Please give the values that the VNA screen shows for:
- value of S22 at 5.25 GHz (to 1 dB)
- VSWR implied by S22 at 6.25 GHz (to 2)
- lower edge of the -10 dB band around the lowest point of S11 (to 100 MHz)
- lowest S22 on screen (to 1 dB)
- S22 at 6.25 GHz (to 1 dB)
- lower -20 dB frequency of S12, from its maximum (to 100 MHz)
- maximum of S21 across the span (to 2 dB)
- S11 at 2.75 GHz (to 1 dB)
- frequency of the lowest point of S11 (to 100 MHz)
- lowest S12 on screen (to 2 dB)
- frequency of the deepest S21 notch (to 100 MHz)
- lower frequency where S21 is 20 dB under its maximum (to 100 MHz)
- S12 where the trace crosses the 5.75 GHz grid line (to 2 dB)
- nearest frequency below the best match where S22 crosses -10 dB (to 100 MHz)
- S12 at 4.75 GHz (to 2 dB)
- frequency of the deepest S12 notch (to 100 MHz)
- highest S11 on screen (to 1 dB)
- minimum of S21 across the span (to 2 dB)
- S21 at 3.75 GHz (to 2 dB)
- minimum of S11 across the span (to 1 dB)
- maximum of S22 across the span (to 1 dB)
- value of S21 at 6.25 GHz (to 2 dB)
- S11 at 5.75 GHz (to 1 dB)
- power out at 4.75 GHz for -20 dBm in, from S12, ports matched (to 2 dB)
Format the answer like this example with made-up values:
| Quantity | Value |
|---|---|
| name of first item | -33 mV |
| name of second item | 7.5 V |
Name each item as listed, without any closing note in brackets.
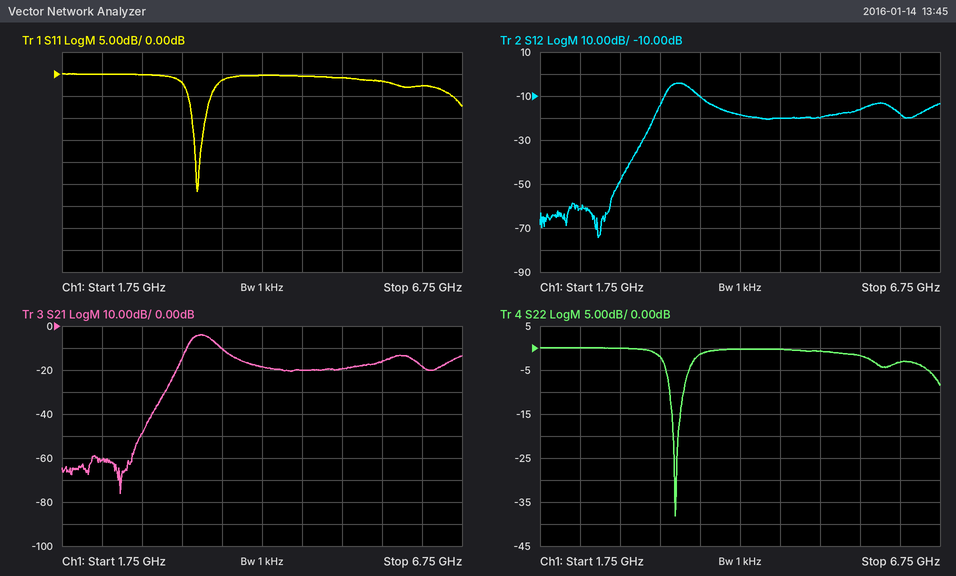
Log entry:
| Quantity | Value |
|---|---|
| value of S22 at 5.25 GHz | -1 dB |
| VSWR implied by S22 at 6.25 GHz | 6 |
| lower edge of the -10 dB band around the lowest point of S11 | 3.4 GHz |
| lowest S22 on screen | -38 dB |
| S22 at 6.25 GHz | -3 dB |
| lower -20 dB frequency of S12, from its maximum | 3.1 GHz |
| maximum of S21 across the span | -4 dB |
| S11 at 2.75 GHz | 0 dB |
| frequency of the lowest point of S11 | 3.4 GHz |
| lowest S12 on screen | -74 dB |
| frequency of the deepest S21 notch | 2.5 GHz |
| lower frequency where S21 is 20 dB under its maximum | 3.1 GHz |
| S12 where the trace crosses the 5.75 GHz grid line | -16 dB |
| nearest frequency below the best match where S22 crosses -10 dB | 3.4 GHz |
| S12 at 4.75 GHz | -20 dB |
| frequency of the deepest S12 notch | 2.5 GHz |
| highest S11 on screen | 0 dB |
| minimum of S21 across the span | -76 dB |
| S21 at 3.75 GHz | -10 dB |
| minimum of S11 across the span | -27 dB |
| maximum of S22 across the span | 0 dB |
| value of S21 at 6.25 GHz | -18 dB |
| S11 at 5.75 GHz | -2 dB |
| power out at 4.75 GHz for -20 dBm in, from S12, ports matched | -40 dBm |
